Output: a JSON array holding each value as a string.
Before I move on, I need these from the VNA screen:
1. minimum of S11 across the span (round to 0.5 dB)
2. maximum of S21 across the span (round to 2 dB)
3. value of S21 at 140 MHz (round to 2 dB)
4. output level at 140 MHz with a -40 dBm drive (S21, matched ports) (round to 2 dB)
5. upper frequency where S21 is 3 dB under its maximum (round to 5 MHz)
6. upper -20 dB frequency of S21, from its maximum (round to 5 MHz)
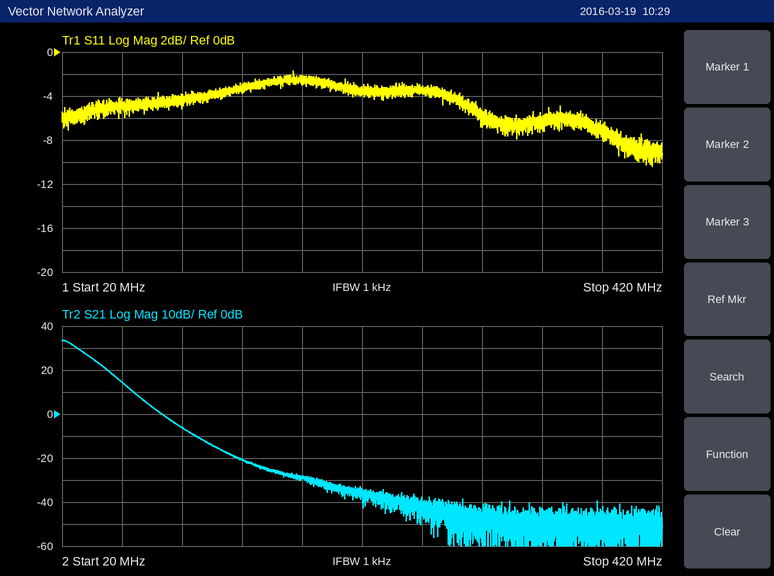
["-10.5 dB", "34 dB", "-20 dB", "-60 dBm", "30 MHz", "60 MHz"]
